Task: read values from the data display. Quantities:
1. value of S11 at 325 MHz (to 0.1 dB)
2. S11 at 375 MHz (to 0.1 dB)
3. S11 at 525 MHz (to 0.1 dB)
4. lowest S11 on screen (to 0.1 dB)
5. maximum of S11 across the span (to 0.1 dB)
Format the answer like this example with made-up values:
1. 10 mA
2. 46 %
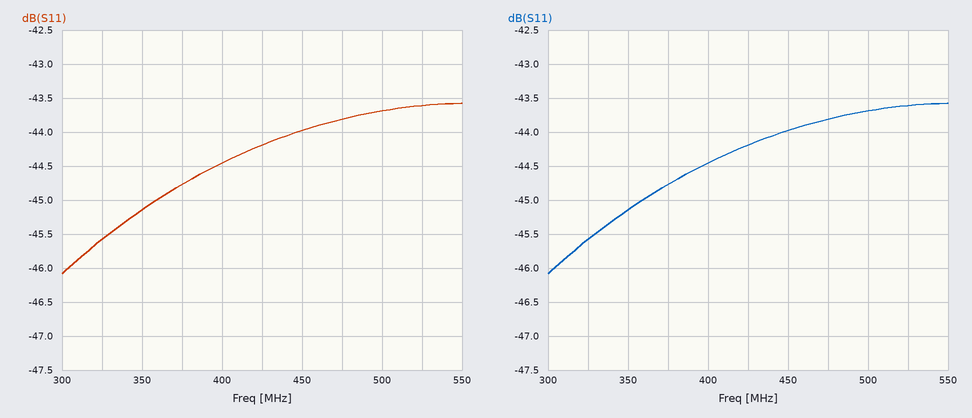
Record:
1. -45.6 dB
2. -44.8 dB
3. -43.6 dB
4. -46.1 dB
5. -43.6 dB
